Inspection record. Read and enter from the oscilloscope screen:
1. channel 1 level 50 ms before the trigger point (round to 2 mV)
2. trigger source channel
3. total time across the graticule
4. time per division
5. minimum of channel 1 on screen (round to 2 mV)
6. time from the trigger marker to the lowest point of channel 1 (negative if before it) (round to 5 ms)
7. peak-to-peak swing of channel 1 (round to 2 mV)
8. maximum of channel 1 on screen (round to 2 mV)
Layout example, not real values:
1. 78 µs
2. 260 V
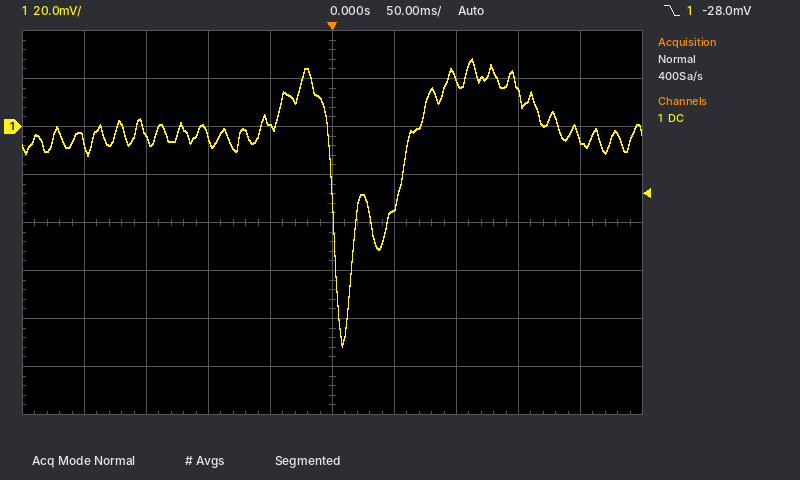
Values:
1. 0 mV
2. channel 1
3. 500 ms
4. 50 ms
5. -92 mV
6. +10 ms
7. 120 mV
8. 28 mV
